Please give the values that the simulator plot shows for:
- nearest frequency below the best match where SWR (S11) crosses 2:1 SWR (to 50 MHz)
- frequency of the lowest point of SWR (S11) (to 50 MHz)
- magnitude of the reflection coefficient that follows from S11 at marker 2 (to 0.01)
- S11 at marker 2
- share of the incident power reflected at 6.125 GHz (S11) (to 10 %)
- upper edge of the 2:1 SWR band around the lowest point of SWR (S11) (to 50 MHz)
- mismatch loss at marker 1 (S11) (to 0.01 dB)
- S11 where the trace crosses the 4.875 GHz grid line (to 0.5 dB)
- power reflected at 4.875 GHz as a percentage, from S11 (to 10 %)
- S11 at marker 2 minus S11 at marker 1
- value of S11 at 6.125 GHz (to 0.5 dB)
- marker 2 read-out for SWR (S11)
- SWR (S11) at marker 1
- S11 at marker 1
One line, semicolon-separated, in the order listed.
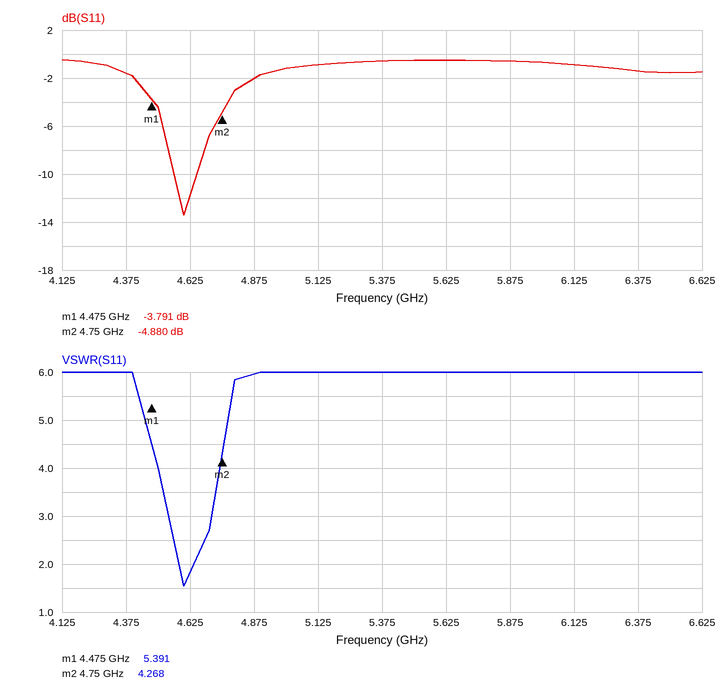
4.60 GHz; 4.60 GHz; 0.57; -4.880 dB; 80 %; 4.65 GHz; 2.35 dB; -2.0 dB; 60 %; -1.089 dB; -1.0 dB; 4.268; 5.391; -3.791 dB
